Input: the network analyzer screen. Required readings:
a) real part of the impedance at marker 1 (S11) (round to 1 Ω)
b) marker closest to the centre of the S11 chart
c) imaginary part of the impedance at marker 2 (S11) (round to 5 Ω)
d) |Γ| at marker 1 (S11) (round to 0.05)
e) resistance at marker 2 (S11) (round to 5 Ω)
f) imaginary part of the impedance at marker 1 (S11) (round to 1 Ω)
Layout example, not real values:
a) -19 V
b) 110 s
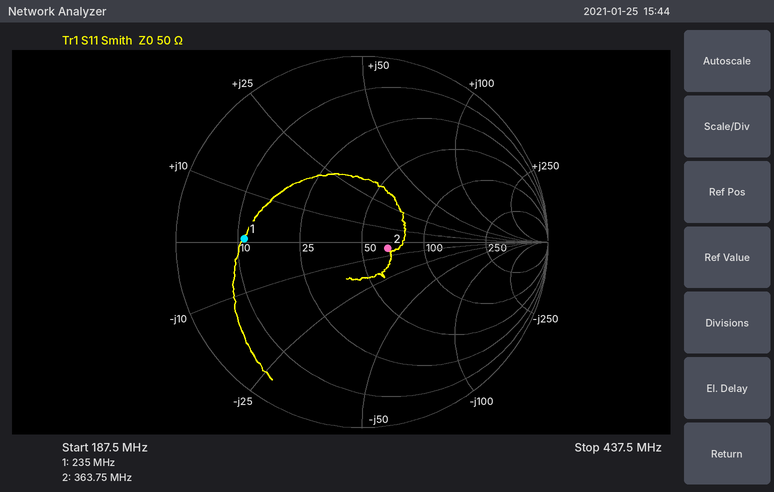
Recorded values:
a) 11 Ω
b) marker 2
c) -5 Ω
d) 0.65
e) 65 Ω
f) +1 Ω
